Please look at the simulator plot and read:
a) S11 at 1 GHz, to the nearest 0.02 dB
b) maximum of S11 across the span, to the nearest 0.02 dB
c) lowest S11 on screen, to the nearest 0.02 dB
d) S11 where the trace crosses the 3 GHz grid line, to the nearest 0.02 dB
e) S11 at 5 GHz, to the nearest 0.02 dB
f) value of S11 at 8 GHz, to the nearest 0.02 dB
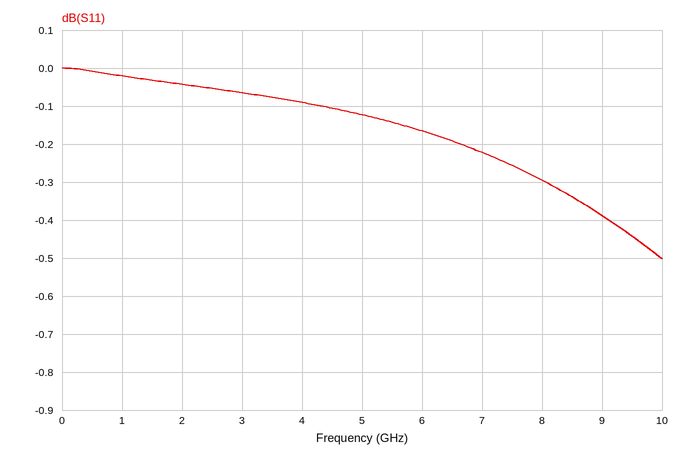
-0.02 dB
0.00 dB
-0.50 dB
-0.06 dB
-0.12 dB
-0.30 dB
